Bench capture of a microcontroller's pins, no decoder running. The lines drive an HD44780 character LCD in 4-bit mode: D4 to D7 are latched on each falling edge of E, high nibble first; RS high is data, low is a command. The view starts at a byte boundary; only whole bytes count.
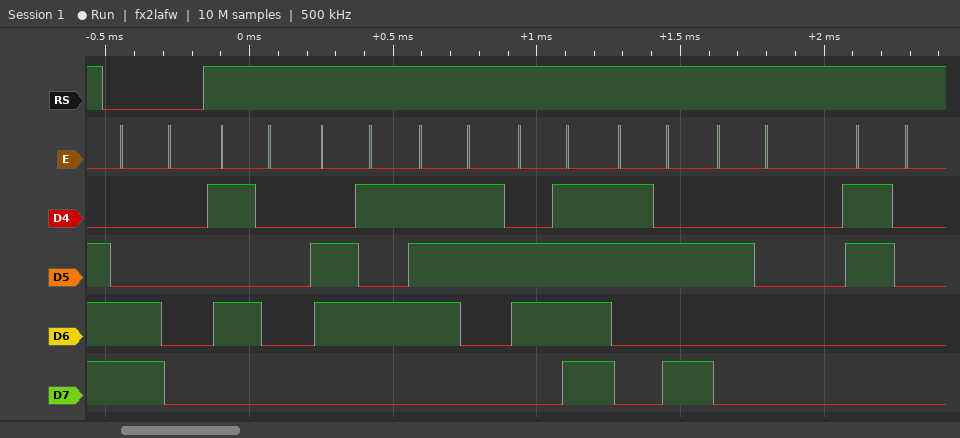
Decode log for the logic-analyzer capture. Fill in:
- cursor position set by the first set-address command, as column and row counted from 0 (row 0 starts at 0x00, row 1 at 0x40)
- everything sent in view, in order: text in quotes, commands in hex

column 0, row 1
0xC0 "Peso: 0"
